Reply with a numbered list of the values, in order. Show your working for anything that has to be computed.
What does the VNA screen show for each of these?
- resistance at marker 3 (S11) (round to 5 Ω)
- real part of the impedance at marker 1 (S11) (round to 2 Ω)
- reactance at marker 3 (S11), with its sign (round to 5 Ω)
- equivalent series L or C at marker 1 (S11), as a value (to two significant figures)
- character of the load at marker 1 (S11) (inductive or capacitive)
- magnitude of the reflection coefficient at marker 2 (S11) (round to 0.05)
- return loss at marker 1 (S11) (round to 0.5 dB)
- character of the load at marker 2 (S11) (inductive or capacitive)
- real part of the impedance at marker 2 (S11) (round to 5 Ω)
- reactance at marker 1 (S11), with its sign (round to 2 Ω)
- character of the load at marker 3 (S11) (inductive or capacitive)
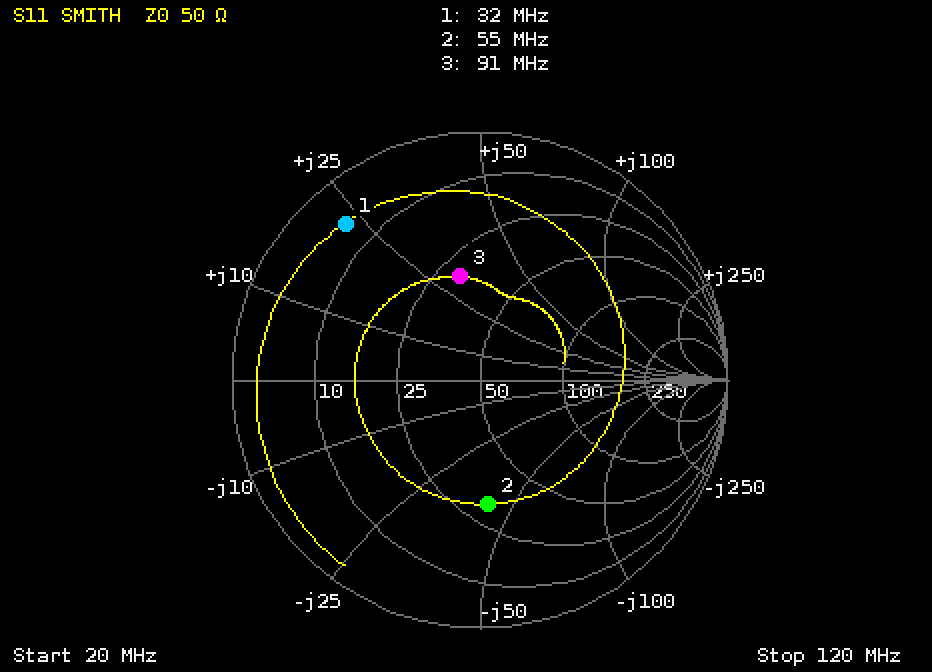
1. 30 Ω
2. 6 Ω
3. +30 Ω
4. L = 22 Ω/(2π × 32 MHz) ≈ 109 nH, so 110 nH to two significant figures
5. inductive
6. 0.50
7. 1.5 dB
8. capacitive
9. 30 Ω
10. +22 Ω
11. inductive
